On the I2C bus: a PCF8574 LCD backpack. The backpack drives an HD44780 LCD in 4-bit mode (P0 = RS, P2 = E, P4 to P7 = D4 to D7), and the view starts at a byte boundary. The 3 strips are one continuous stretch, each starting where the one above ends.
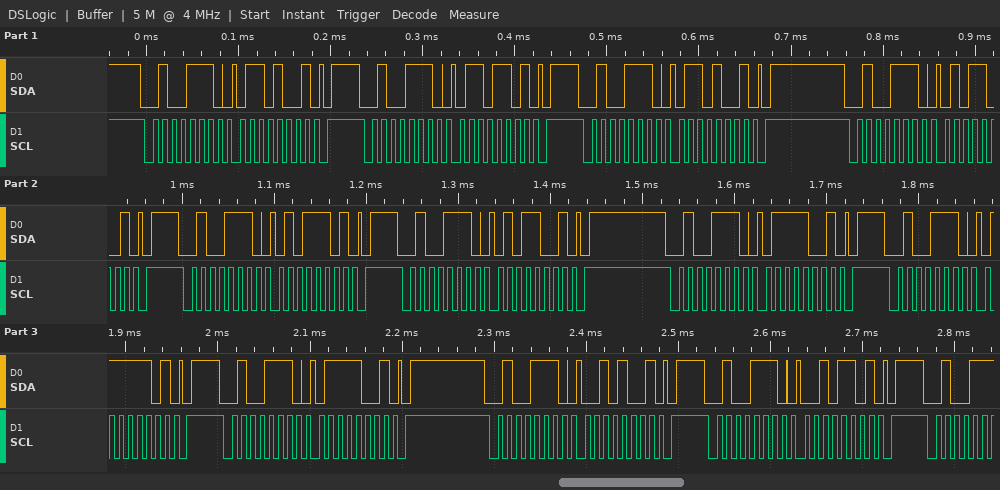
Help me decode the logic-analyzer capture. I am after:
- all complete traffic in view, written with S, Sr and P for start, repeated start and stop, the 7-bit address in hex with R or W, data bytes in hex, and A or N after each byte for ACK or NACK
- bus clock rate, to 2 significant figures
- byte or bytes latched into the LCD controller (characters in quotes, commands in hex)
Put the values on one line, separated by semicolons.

S 27W A 69 A P S 27W A 6D A P S 27W A 69 A P S 27W A 59 A P S 27W A 5D A P S 27W A 59 A P S 27W A 79 A P S 27W A 7D A P S 27W A 79 A P S 27W A 29 A P S 27W A 2D A P; 100 kHz; 'e'
